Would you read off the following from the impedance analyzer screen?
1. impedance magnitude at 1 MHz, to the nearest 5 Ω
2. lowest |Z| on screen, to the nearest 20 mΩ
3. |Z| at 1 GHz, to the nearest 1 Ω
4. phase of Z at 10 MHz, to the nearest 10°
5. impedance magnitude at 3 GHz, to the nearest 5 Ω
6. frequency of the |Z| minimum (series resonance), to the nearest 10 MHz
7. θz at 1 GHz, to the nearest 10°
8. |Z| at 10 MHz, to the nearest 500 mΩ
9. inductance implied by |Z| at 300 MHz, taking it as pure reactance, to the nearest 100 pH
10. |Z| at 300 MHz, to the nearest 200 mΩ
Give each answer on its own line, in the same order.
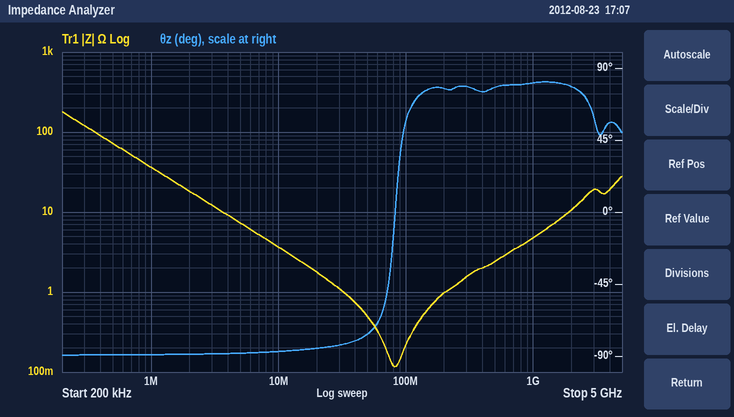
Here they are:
35 Ω
120 mΩ
5 Ω
-90°
20 Ω
80 MHz
80°
3.5 Ω
800 pH
1.6 Ω
